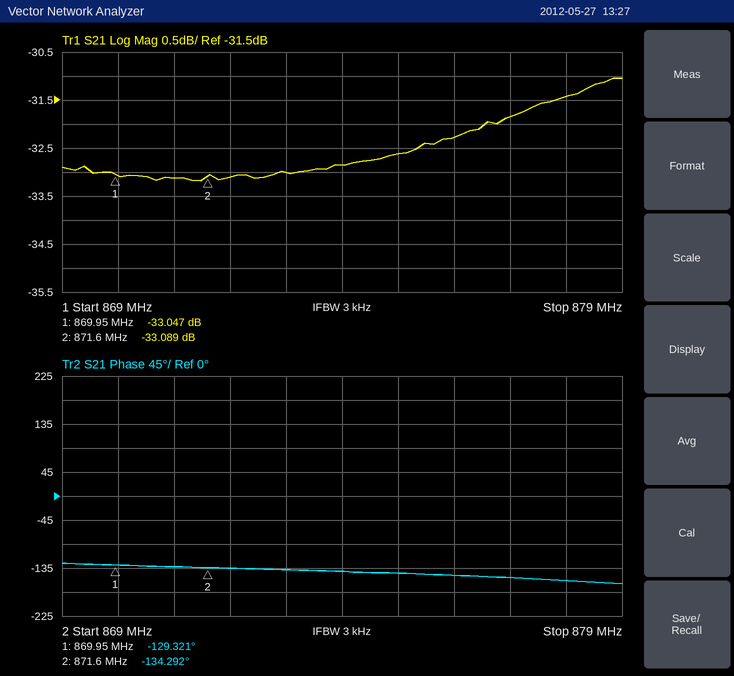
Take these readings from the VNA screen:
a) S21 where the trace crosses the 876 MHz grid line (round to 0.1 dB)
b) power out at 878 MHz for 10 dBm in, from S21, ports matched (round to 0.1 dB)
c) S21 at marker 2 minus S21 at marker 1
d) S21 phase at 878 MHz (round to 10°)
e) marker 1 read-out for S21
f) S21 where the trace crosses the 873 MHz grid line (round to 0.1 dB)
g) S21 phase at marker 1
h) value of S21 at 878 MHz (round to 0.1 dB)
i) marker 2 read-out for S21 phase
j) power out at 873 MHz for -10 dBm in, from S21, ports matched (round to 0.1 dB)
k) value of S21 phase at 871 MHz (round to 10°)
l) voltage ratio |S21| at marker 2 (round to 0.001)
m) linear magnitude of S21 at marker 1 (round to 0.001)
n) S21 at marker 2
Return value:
-32.3 dB
-21.4 dBm
-0.042 dB
-160°
-33.047 dB
-33.0 dB
-129.321°
-31.4 dB
-134.292°
-43.0 dBm
-130°
0.022
0.022
-33.089 dB
